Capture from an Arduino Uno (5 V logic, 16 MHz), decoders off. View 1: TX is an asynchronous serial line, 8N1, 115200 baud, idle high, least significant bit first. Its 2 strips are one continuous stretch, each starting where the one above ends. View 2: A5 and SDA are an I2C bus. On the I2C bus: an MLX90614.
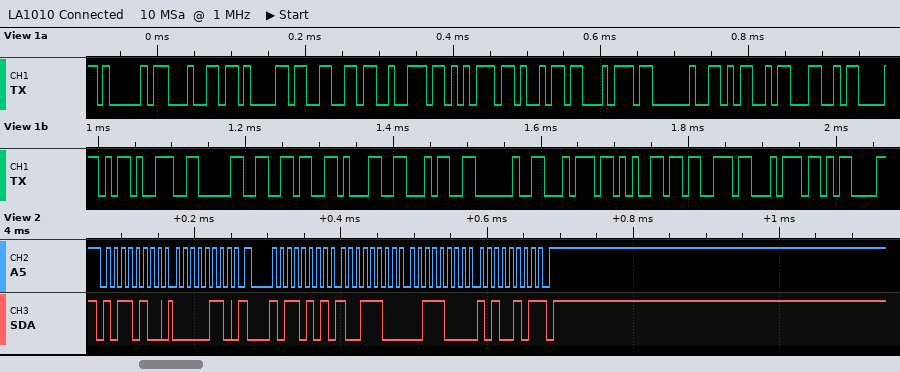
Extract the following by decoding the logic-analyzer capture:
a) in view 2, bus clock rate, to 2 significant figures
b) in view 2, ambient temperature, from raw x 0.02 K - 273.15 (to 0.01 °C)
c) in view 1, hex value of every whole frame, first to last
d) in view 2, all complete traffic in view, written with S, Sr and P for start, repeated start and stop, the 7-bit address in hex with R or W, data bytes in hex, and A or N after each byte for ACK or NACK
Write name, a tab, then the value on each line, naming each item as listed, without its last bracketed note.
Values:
in view 2, bus clock rate, to 2 significant figures	100 kHz
in view 2, ambient temperature, from raw x 0.02 K - 273.15	16.69 °C
in view 1, hex value of every whole frame, first to last	0x41 0x64 0x61 0x66 0x72 0x75 0x69 0x74 0x20 0x4D 0x4C 0x58 0x39 0x30 0x36 0x31 0x34 0x20 0x74 0x65 0x73 0x74 0x0D
in view 2, all complete traffic in view, written with S, Sr and P for start, repeated start and stop, the 7-bit address in hex with R or W, data bytes in hex, and A or N after each byte for ACK or NACK	S 5AW A 06 A Sr 5AR A 9C A 38 A A5 N P
